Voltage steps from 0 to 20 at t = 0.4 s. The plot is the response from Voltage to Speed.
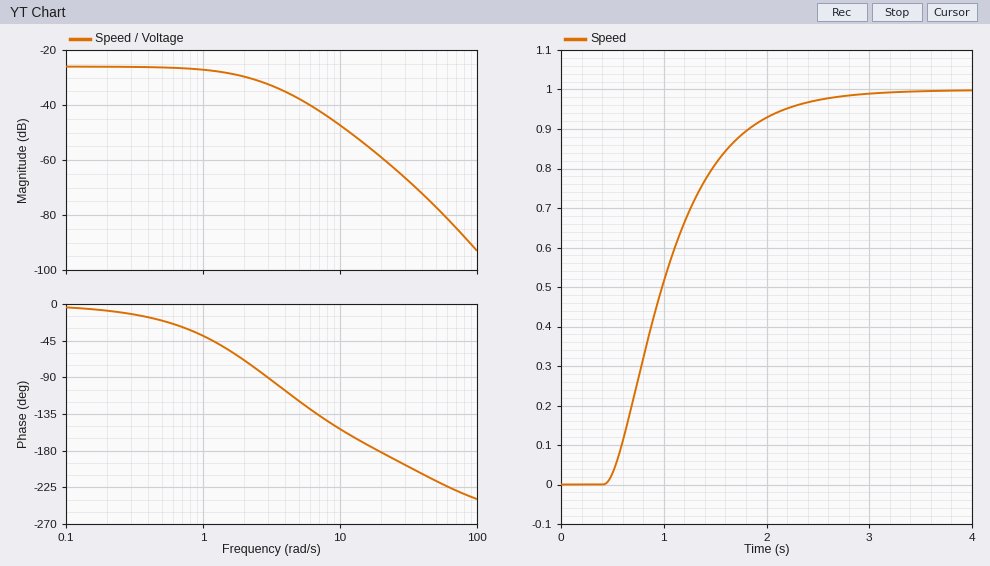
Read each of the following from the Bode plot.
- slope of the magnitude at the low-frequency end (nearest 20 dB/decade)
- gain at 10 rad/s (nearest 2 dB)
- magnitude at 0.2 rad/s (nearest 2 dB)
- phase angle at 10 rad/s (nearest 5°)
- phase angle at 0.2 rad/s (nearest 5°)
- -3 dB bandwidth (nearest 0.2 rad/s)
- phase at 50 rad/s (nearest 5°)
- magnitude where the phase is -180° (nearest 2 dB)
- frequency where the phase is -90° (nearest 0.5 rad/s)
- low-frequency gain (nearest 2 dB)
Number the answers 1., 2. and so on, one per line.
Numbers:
1. 0 dB/decade
2. -48 dB
3. -26 dB
4. -155°
5. -10°
6. 1.8 rad/s
7. -215°
8. -58 dB
9. 3.0 rad/s
10. -26 dB
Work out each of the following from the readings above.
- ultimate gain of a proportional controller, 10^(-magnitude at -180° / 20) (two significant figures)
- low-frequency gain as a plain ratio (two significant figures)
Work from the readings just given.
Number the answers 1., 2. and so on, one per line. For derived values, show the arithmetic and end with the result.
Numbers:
1. 10^(58 / 20) = 790
2. 10^(-26 / 20) = 0.050
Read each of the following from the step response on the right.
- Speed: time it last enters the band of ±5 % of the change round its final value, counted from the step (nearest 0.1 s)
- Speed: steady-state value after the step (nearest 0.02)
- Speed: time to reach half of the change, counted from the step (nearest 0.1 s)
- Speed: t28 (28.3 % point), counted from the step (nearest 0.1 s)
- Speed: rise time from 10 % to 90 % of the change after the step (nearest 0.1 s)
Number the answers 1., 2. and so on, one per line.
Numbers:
1. 1.8 s
2. 1.00
3. 0.6 s
4. 0.4 s
5. 1.2 s
